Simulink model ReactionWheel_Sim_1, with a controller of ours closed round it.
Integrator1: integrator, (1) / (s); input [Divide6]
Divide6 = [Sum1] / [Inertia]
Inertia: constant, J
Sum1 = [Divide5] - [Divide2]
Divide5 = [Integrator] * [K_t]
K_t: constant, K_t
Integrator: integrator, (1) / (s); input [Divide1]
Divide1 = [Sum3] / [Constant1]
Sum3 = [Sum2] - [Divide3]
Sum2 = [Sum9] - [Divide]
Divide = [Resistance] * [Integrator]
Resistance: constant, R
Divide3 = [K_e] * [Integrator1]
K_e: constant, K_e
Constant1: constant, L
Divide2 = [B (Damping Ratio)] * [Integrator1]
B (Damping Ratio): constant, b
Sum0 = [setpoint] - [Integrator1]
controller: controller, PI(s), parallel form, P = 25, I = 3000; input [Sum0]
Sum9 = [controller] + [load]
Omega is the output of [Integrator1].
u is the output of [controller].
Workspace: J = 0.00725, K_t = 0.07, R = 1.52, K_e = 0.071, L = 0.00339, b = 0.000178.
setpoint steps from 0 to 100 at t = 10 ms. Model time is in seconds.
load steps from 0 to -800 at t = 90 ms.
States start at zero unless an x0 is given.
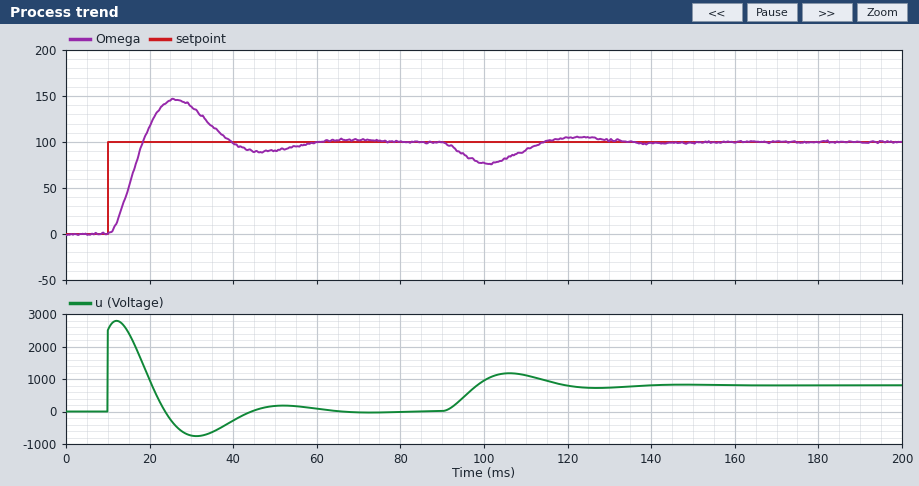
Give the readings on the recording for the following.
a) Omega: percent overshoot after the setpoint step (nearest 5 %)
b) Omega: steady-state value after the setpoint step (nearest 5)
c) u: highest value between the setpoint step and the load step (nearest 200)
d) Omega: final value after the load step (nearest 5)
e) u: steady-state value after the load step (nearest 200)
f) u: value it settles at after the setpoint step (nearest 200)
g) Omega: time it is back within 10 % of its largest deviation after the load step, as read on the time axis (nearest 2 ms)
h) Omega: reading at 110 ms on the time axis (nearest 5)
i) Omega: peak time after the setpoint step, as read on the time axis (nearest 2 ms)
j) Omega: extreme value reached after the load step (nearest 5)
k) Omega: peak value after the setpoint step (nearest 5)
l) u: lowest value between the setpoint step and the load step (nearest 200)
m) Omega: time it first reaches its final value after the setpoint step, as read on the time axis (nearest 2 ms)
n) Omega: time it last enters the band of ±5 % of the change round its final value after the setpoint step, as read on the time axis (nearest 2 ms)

45 %
100
2800
100
800
0
130 ms
90
26 ms
75
145
-800
18 ms
54 ms
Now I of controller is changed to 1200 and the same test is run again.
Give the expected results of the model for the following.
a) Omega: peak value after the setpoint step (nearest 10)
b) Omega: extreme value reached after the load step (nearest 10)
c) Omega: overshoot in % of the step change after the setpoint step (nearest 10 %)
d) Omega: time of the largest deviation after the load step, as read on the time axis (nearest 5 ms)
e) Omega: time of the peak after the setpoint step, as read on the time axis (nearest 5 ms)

120
70
20 %
105 ms
30 ms
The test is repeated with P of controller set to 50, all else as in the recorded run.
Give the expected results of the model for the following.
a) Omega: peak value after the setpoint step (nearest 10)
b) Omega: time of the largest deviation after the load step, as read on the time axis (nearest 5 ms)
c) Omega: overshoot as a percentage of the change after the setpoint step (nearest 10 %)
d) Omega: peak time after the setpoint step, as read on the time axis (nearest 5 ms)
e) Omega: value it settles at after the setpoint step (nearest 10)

130
100 ms
30 %
20 ms
100
